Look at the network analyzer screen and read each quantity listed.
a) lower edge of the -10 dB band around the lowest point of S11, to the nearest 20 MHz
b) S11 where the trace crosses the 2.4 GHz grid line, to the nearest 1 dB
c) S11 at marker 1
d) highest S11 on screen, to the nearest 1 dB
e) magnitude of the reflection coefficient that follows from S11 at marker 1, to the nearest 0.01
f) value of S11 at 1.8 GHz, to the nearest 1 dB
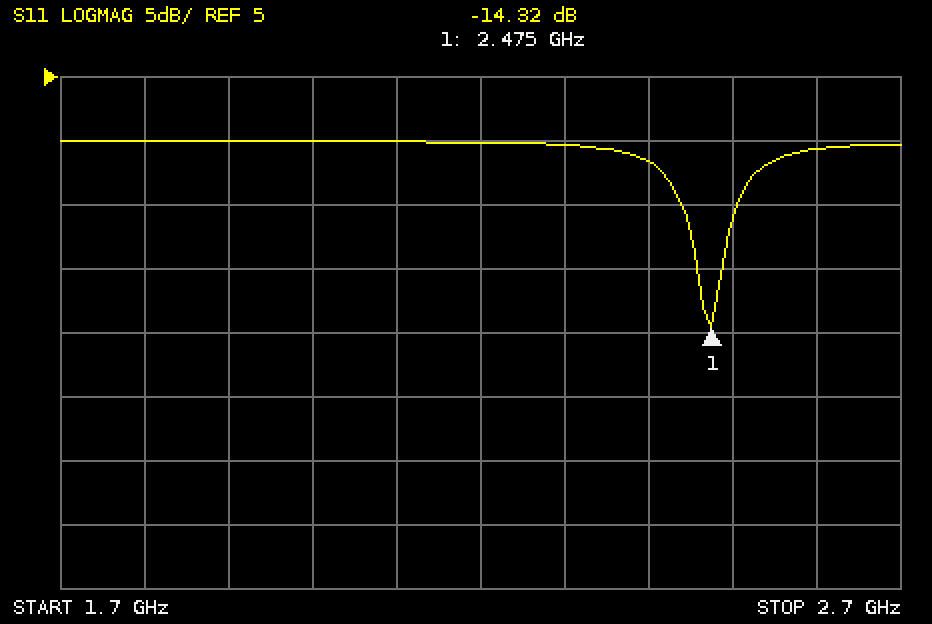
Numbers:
2.46 GHz
-2 dB
-14.32 dB
0 dB
0.19
0 dB
